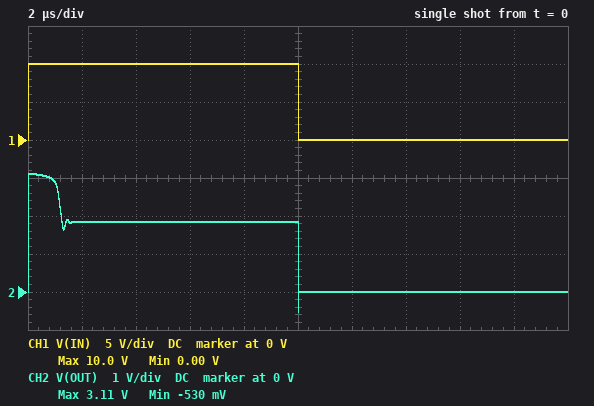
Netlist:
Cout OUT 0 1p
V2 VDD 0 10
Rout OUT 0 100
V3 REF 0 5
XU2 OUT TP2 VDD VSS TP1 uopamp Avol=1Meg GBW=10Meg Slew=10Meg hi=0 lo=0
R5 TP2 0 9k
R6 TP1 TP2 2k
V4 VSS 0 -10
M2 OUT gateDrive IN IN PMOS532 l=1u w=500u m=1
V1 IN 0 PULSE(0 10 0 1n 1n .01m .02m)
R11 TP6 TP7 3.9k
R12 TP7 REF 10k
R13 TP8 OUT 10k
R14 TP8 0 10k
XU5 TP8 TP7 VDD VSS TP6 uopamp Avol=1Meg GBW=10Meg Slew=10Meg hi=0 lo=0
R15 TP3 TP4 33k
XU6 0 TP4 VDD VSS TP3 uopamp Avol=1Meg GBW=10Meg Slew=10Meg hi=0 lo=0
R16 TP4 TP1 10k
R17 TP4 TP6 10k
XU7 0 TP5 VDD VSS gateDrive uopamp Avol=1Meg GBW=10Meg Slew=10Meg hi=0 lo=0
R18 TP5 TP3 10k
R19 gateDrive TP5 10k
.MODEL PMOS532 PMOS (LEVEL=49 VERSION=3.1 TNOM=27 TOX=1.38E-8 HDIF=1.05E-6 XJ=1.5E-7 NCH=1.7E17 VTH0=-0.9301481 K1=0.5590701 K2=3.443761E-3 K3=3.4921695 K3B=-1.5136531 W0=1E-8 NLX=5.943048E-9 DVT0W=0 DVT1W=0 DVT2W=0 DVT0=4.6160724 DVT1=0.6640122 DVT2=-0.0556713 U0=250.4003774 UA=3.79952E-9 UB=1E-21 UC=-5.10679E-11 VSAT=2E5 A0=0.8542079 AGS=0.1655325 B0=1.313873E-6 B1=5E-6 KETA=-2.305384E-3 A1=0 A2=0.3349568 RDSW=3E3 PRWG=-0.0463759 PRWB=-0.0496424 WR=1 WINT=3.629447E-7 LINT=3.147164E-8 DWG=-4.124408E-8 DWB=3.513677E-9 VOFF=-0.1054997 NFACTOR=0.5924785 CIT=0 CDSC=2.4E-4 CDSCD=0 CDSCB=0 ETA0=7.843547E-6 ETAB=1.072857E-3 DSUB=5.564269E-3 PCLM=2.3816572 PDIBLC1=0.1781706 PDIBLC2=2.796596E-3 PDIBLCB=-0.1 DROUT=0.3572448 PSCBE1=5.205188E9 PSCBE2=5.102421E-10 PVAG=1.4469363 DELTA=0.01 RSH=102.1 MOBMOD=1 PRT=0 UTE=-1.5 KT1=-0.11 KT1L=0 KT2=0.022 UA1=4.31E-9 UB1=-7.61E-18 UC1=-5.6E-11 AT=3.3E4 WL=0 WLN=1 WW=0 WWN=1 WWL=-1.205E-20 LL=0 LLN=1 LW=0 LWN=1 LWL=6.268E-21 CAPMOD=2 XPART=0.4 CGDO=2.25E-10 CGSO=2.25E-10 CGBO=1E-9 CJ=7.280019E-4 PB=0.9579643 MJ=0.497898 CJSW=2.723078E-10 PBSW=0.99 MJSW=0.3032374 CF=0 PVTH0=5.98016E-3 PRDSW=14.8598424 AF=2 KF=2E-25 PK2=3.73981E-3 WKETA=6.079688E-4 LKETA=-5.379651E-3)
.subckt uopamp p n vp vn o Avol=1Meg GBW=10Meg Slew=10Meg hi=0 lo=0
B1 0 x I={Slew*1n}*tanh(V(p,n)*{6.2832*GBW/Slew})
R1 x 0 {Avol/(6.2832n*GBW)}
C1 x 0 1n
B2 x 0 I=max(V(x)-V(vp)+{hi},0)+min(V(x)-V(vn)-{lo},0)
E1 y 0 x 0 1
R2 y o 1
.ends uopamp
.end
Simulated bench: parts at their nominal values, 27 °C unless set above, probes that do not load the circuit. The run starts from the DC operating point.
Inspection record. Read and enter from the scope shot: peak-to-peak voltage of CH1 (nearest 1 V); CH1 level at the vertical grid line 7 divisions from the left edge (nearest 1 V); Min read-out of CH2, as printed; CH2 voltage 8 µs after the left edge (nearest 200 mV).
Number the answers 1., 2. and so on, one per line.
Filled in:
1. 10 V
2. 0 V
3. -530 mV
4. 1.8 V
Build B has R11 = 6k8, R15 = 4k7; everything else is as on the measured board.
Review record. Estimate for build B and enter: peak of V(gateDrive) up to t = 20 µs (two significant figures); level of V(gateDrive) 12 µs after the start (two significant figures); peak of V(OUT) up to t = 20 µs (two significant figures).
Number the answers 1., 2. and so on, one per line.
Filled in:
1. 1.3 V
2. -1.6 V
3. 3.1 V
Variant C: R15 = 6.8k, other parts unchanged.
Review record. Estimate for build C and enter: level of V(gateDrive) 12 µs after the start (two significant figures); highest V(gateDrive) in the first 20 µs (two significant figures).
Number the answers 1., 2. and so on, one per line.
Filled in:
1. -1.3 V
2. 2.5 V
